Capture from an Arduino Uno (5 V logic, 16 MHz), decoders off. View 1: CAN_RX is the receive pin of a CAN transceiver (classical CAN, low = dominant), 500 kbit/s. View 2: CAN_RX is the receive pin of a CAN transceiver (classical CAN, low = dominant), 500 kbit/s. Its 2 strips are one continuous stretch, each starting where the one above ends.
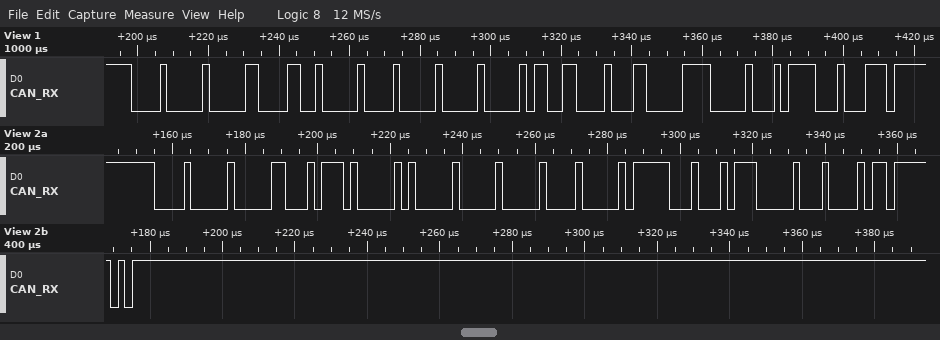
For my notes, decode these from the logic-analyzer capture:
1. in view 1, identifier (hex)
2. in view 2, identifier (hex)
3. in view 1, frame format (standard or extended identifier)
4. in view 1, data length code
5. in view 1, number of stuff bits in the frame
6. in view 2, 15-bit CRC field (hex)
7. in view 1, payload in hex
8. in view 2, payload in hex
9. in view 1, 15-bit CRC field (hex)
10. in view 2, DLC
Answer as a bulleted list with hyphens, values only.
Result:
- 0x080
- 0x080
- standard
- 8
- 8
- 0x42DF
- 64 01 00 00 CC 23 07 00
- BA 04 00 00 40 F9 17 00
- 0x5E23
- 8
